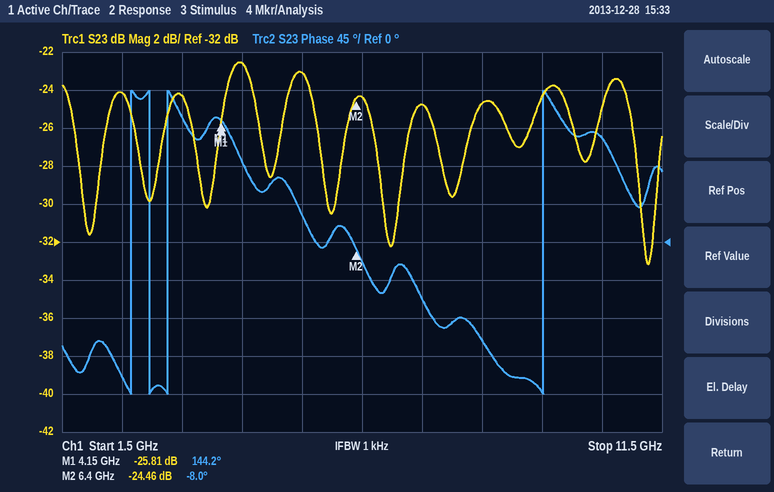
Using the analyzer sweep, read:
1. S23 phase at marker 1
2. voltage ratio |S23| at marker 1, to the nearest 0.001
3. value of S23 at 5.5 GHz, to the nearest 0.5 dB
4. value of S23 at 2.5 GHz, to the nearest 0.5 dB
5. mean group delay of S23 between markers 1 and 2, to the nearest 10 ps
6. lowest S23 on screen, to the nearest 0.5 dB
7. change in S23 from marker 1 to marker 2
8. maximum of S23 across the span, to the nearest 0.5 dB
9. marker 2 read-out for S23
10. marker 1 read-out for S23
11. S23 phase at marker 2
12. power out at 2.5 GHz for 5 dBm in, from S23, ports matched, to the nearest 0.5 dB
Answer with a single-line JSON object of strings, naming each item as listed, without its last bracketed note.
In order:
{"S23 phase at marker 1": "144.2°", "voltage ratio |S23| at marker 1, to the nearest 0.001": "0.051", "value of S23 at 5.5 GHz, to the nearest 0.5 dB": "-23.0 dB", "value of S23 at 2.5 GHz, to the nearest 0.5 dB": "-24.0 dB", "mean group delay of S23 between markers 1 and 2, to the nearest 10 ps": "190 ps", "lowest S23 on screen, to the nearest 0.5 dB": "-33.0 dB", "change in S23 from marker 1 to marker 2": "1.35 dB", "maximum of S23 across the span, to the nearest 0.5 dB": "-22.5 dB", "marker 2 read-out for S23": "-24.46 dB", "marker 1 read-out for S23": "-25.81 dB", "S23 phase at marker 2": "-8.0°", "power out at 2.5 GHz for 5 dBm in, from S23, ports matched, to the nearest 0.5 dB": "-19.0 dBm"}
